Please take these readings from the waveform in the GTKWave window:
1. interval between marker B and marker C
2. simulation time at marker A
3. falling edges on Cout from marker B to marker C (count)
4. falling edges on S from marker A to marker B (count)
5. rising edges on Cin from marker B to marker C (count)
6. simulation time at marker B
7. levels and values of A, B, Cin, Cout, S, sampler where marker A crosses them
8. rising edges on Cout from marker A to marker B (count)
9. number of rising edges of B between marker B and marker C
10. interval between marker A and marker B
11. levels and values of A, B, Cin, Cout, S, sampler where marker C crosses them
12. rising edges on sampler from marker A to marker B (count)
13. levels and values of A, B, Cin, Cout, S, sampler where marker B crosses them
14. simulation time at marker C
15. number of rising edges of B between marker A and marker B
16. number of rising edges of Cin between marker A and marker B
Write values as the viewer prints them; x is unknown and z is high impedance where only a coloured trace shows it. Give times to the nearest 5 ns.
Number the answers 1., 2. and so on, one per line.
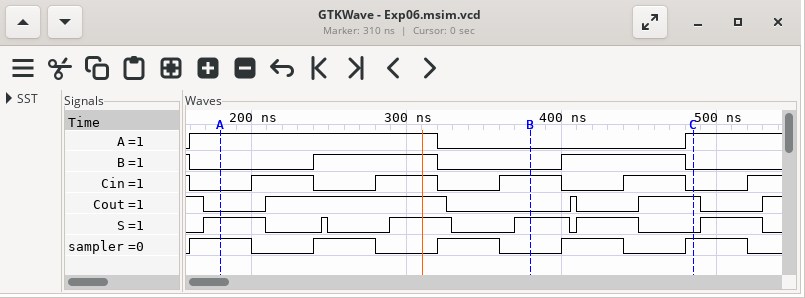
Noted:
1. 105 ns
2. 180 ns
3. 1
4. 3
5. 1
6. 380 ns
7. A=1, B=0, Cin=0, Cout=0, S=1, sampler=1
8. 1
9. 1
10. 200 ns
11. A=1, B=0, Cin=0, Cout=1, S=0, sampler=1
12. 2
13. A=0, B=0, Cin=1, Cout=0, S=1, sampler=0
14. 485 ns
15. 1
16. 3
